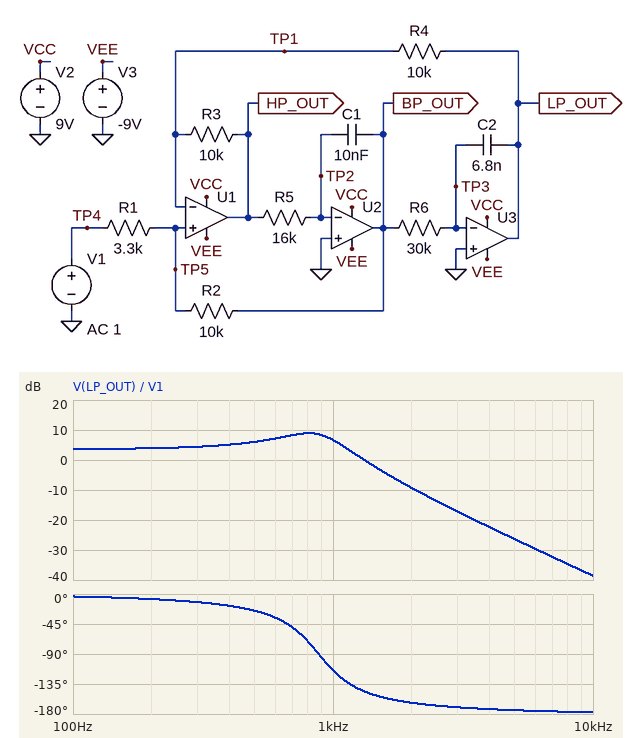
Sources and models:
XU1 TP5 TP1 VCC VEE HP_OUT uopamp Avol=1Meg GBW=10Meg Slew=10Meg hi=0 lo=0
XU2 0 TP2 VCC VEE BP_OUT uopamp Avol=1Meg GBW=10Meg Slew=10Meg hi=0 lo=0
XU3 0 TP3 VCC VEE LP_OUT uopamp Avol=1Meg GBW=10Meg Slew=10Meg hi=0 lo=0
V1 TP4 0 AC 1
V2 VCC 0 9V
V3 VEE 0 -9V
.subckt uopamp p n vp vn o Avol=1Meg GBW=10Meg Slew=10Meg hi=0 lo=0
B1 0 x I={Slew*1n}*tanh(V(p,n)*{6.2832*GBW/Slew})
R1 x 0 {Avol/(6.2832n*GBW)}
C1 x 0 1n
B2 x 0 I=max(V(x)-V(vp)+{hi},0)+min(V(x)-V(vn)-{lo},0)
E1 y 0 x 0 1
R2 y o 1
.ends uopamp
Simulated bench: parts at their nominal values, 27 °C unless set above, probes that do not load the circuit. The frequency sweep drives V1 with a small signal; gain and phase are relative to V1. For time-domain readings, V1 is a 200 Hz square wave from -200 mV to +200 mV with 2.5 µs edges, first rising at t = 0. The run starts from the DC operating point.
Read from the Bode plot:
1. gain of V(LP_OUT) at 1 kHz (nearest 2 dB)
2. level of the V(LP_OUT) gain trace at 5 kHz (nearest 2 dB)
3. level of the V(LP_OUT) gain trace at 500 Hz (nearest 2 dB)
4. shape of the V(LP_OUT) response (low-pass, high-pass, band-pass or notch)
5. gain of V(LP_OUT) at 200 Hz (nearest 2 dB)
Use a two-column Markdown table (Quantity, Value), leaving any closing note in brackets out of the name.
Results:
| Quantity | Value |
|---|---|
| gain of V(LP_OUT) at 1 kHz | 6 dB |
| level of the V(LP_OUT) gain trace at 5 kHz | -26 dB |
| level of the V(LP_OUT) gain trace at 500 Hz | 6 dB |
| shape of the V(LP_OUT) response | low-pass |
| gain of V(LP_OUT) at 200 Hz | 4 dB |
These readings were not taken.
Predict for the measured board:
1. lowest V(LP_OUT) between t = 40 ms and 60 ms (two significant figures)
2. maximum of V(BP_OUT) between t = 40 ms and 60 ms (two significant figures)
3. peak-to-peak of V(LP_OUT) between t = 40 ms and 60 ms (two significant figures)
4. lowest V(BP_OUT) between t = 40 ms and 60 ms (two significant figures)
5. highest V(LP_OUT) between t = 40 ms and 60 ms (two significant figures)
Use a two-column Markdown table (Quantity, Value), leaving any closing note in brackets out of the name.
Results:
| Quantity | Value |
|---|---|
| lowest V(LP_OUT) between t = 40 ms and 60 ms | -540 mV |
| maximum of V(BP_OUT) between t = 40 ms and 60 ms | 460 mV |
| peak-to-peak of V(LP_OUT) between t = 40 ms and 60 ms | 1.1 V |
| lowest V(BP_OUT) between t = 40 ms and 60 ms | -460 mV |
| highest V(LP_OUT) between t = 40 ms and 60 ms | 540 mV |
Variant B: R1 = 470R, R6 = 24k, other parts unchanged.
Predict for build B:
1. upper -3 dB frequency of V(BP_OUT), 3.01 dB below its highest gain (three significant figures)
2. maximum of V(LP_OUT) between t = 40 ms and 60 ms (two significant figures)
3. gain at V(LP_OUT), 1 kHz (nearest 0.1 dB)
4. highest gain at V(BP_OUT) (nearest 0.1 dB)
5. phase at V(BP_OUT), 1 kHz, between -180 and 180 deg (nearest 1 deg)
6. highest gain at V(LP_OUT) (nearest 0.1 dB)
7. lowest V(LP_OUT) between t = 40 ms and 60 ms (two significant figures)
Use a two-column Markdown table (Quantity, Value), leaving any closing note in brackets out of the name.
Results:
| Quantity | Value |
|---|---|
| upper -3 dB frequency of V(BP_OUT), 3.01 dB below its highest gain | 1.03 kHz |
| maximum of V(LP_OUT) between t = 40 ms and 60 ms | 1.6 V |
| gain at V(LP_OUT), 1 kHz | 25.9 dB |
| highest gain at V(BP_OUT) | 26.6 dB |
| phase at V(BP_OUT), 1 kHz, between -180 and 180 deg | 161 deg |
| highest gain at V(LP_OUT) | 26.5 dB |
| lowest V(LP_OUT) between t = 40 ms and 60 ms | -1.6 V |
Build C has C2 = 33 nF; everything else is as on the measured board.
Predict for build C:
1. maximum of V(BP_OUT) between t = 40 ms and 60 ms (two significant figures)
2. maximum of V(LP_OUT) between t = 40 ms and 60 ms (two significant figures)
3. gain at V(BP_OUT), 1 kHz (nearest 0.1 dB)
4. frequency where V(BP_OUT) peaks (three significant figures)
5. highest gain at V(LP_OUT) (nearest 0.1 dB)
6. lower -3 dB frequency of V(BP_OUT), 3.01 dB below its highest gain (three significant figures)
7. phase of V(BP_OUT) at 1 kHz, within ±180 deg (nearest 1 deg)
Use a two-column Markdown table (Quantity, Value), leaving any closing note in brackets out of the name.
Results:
| Quantity | Value |
|---|---|
| maximum of V(BP_OUT) between t = 40 ms and 60 ms | 740 mV |
| maximum of V(LP_OUT) between t = 40 ms and 60 ms | 350 mV |
| gain at V(BP_OUT), 1 kHz | 3.7 dB |
| frequency where V(BP_OUT) peaks | 400 Hz |
| highest gain at V(LP_OUT) | 3.8 dB |
| lower -3 dB frequency of V(BP_OUT), 3.01 dB below its highest gain | 223 Hz |
| phase of V(BP_OUT) at 1 kHz, within ±180 deg | 120 deg |
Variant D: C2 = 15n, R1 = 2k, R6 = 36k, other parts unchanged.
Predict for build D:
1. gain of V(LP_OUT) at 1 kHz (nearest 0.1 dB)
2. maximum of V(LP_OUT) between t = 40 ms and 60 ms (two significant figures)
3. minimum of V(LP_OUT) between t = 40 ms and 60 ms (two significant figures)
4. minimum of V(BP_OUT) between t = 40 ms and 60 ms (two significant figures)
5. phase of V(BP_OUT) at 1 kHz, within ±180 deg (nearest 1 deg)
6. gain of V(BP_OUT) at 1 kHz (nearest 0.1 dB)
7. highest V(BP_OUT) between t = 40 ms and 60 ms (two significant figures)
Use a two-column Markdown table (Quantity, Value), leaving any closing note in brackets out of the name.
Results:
| Quantity | Value |
|---|---|
| gain of V(LP_OUT) at 1 kHz | -4.1 dB |
| maximum of V(LP_OUT) between t = 40 ms and 60 ms | 570 mV |
| minimum of V(LP_OUT) between t = 40 ms and 60 ms | -570 mV |
| minimum of V(BP_OUT) between t = 40 ms and 60 ms | -810 mV |
| phase of V(BP_OUT) at 1 kHz, within ±180 deg | 115 deg |
| gain of V(BP_OUT) at 1 kHz | 6.5 dB |
| highest V(BP_OUT) between t = 40 ms and 60 ms | 810 mV |
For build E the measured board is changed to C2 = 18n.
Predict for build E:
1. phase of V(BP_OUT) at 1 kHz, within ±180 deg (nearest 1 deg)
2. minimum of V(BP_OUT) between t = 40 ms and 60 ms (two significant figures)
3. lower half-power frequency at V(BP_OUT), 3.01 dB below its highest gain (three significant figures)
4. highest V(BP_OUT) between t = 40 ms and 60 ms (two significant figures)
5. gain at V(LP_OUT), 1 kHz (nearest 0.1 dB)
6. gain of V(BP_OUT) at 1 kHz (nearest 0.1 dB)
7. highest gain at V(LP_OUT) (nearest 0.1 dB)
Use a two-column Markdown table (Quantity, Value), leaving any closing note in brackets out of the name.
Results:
| Quantity | Value |
|---|---|
| phase of V(BP_OUT) at 1 kHz, within ±180 deg | 125 deg |
| minimum of V(BP_OUT) between t = 40 ms and 60 ms | -620 mV |
| lower half-power frequency at V(BP_OUT), 3.01 dB below its highest gain | 348 Hz |
| highest V(BP_OUT) between t = 40 ms and 60 ms | 620 mV |
| gain at V(LP_OUT), 1 kHz | -5.8 dB |
| gain of V(BP_OUT) at 1 kHz | 4.8 dB |
| highest gain at V(LP_OUT) | 5.4 dB |
